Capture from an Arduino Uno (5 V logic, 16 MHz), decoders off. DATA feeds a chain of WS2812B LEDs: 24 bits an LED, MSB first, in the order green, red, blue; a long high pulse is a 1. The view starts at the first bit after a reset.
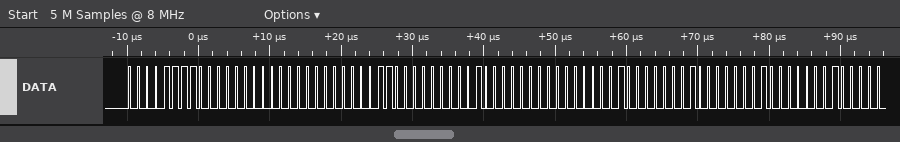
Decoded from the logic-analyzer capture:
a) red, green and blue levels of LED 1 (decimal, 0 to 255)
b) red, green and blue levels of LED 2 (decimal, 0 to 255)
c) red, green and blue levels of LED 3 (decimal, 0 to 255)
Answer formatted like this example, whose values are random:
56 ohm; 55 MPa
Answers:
0, 15, 0; 1, 12, 0; 1, 1, 1
